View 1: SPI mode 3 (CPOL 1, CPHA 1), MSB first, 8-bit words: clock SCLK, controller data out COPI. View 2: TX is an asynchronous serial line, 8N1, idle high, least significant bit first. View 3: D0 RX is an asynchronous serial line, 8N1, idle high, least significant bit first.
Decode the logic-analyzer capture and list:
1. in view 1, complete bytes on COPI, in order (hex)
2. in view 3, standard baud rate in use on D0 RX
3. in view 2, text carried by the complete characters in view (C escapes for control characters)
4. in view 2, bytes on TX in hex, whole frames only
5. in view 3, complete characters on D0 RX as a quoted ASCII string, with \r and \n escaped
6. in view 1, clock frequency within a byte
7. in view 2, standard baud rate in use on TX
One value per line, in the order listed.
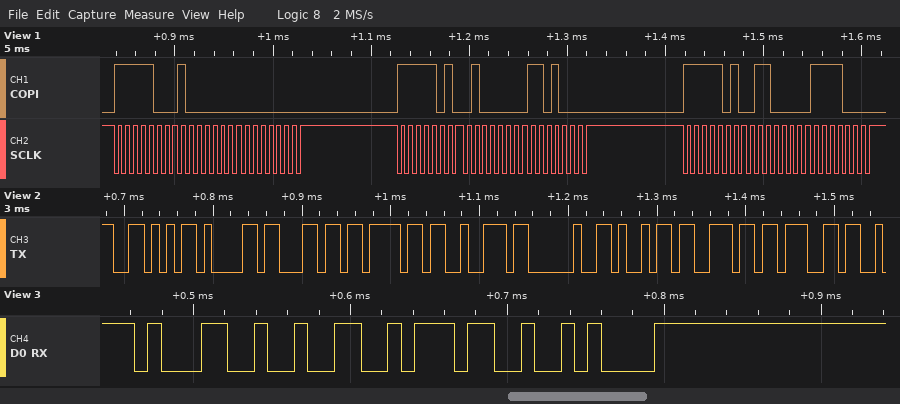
F8 80 00 FA 40 D0 FA 60 F0
115200 baud
"Valor ing"
56 61 6C 6F 72 20 69 6E 67
"127\n"
125 kHz
115200 baud
